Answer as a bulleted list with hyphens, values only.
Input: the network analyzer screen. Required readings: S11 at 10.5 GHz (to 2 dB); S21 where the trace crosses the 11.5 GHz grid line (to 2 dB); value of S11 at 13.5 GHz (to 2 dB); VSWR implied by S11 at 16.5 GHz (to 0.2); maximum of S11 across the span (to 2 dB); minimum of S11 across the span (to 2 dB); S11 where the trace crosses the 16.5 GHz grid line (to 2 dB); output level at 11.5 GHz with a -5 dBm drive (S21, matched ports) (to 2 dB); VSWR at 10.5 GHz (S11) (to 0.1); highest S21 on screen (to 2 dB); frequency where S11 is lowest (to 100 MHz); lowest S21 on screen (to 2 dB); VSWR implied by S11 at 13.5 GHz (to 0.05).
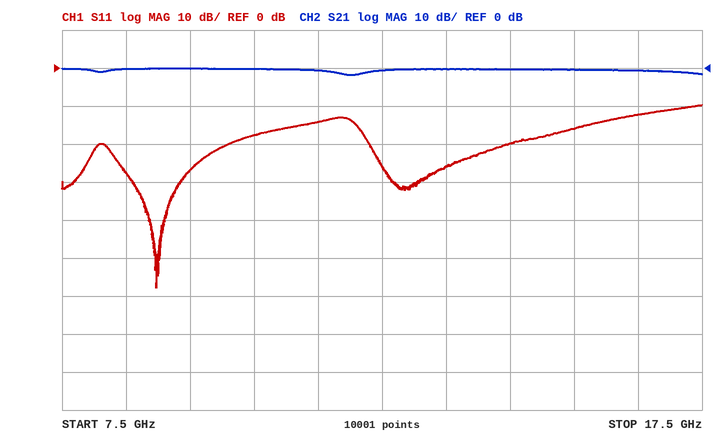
- -18 dB
- 0 dB
- -26 dB
- 1.6
- -10 dB
- -58 dB
- -12 dB
- -6 dBm
- 1.3
- 0 dB
- 9.0 GHz
- -2 dB
- 1.10
